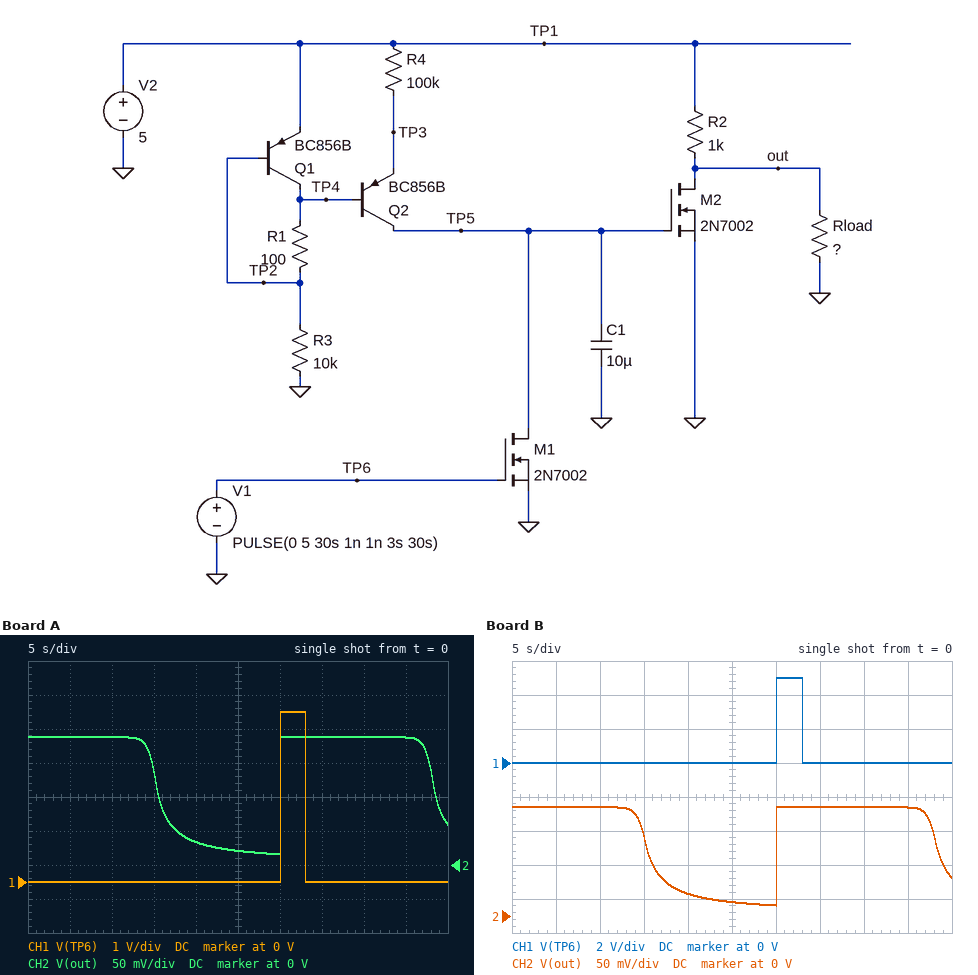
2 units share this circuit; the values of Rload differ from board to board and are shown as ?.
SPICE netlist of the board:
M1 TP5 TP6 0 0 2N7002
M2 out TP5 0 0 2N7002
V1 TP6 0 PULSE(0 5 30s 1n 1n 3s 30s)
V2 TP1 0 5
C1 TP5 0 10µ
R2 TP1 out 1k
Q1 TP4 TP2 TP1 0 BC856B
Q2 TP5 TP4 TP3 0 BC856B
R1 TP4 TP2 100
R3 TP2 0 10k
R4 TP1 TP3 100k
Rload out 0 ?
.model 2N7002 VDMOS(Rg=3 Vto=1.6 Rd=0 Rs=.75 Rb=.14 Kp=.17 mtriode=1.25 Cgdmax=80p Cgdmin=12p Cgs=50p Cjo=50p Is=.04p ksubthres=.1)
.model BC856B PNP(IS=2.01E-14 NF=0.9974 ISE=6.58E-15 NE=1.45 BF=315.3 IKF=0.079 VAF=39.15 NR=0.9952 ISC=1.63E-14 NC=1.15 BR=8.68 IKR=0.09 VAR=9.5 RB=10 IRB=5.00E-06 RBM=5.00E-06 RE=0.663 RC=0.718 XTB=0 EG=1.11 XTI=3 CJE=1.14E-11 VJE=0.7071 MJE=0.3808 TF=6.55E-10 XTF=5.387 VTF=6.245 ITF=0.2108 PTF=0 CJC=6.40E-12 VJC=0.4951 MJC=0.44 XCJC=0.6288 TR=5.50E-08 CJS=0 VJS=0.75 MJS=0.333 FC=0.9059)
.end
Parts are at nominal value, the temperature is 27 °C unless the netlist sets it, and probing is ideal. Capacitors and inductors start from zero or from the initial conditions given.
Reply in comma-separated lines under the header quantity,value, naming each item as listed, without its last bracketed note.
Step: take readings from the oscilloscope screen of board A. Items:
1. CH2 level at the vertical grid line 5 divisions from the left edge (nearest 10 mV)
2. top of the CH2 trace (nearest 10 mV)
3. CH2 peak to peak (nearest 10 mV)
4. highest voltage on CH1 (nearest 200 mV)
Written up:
quantity,value
CH2 level at the vertical grid line 5 divisions from the left edge,20 mV
top of the CH2 trace,190 mV
CH2 peak to peak,170 mV
highest voltage on CH1,5.0 V
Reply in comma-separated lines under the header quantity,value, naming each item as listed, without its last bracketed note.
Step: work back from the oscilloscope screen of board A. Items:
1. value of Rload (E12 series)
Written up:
quantity,value
value of Rload,39 Ω
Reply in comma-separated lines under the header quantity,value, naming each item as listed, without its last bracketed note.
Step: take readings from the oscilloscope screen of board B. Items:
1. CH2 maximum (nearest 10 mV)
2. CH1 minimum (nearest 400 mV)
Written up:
quantity,value
CH2 maximum,160 mV
CH1 minimum,0 V
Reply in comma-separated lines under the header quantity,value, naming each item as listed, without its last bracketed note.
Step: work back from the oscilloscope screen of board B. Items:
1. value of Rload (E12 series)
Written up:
quantity,value
value of Rload,33 Ω
